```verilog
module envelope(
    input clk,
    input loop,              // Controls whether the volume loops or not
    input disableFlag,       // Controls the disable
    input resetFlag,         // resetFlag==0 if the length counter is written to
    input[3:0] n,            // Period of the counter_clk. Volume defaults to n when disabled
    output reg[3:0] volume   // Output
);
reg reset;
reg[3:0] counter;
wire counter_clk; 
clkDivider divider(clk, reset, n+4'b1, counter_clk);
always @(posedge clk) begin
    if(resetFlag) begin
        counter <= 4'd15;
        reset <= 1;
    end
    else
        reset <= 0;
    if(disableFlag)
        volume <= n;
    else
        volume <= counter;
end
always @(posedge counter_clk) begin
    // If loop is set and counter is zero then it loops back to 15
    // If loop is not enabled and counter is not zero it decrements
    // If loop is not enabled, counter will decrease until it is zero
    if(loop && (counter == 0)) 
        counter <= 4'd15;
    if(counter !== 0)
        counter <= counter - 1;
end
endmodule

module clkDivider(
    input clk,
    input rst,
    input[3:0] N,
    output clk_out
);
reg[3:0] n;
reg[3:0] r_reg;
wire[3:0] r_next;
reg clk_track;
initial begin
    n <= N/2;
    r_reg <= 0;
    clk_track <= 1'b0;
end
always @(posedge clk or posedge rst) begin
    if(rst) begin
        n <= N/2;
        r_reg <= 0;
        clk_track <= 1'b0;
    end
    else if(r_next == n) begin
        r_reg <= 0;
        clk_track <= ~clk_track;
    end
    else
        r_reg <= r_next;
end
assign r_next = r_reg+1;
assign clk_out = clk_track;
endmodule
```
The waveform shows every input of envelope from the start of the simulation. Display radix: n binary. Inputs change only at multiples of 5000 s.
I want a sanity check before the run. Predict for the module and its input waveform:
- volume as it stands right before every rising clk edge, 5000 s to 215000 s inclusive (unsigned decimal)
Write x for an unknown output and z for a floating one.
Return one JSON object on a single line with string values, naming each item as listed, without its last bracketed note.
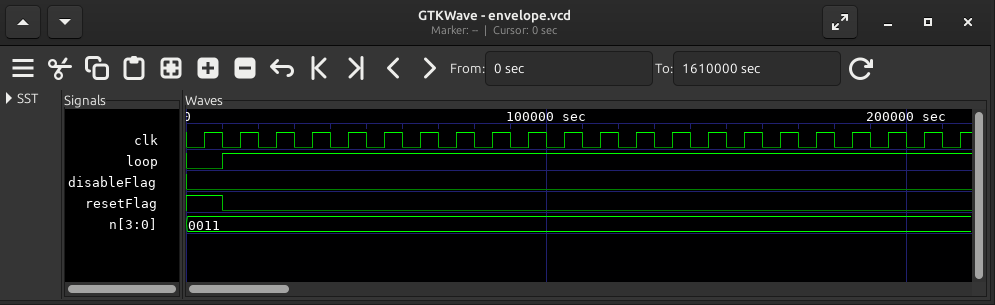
{"volume as it stands right before every rising clk edge, 5000 s to 215000 s inclusive": "x, x, 15, 15, 15, 14, 14, 14, 14, 13, 13, 13, 13, 12, 12, 12, 12, 11, 11, 11, 11, 10"}
